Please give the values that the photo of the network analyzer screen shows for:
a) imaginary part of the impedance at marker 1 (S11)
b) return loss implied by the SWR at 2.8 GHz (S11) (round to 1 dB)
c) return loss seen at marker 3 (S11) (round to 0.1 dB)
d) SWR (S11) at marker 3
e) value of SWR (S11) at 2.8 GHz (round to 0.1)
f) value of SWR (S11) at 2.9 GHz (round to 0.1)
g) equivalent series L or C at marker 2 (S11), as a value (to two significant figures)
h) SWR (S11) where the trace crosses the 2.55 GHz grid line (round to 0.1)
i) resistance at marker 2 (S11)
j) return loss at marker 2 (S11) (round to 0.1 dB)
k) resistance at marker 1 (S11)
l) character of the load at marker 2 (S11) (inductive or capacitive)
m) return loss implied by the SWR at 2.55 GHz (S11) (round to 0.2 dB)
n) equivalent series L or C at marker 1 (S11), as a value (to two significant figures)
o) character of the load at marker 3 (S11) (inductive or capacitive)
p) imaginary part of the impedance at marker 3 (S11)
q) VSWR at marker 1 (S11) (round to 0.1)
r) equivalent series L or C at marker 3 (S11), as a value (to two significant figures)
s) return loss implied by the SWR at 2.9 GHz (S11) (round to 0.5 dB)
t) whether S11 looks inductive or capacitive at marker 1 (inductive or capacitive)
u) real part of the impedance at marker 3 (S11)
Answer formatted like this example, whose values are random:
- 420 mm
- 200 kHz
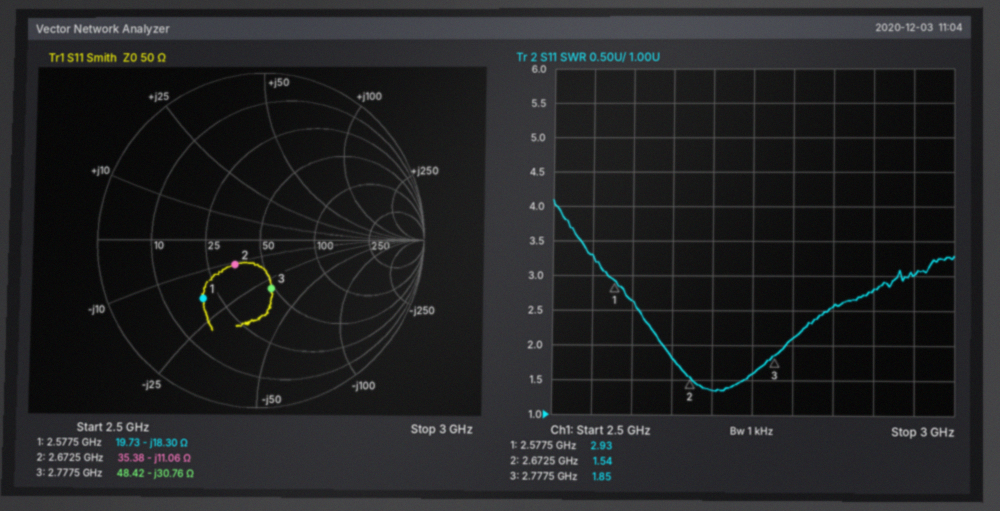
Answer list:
- -18.30 Ω
- 9 dB
- 10.5 dB
- 1.85
- 2.1
- 2.8
- 5.4 pF
- 3.3
- 35.38 Ω
- 13.4 dB
- 19.73 Ω
- capacitive
- 5.4 dB
- 3.4 pF
- capacitive
- -30.76 Ω
- 2.9
- 1.9 pF
- 6.5 dB
- capacitive
- 48.42 Ω
